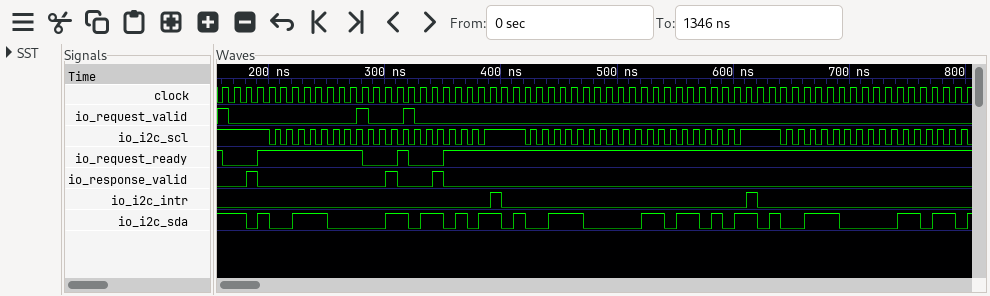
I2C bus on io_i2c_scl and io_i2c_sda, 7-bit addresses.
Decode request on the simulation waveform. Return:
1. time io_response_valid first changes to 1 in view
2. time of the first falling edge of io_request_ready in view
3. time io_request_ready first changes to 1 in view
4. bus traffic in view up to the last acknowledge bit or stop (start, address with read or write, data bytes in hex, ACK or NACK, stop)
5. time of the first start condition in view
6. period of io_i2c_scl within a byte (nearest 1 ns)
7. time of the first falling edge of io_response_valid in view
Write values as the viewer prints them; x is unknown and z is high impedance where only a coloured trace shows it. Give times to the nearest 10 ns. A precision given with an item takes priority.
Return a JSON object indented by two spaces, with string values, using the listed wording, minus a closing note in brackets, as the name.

{
  "time io_response_valid first changes to 1 in view": "180 ns",
  "time of the first falling edge of io_request_ready in view": "160 ns",
  "time io_request_ready first changes to 1 in view": "190 ns",
  "bus traffic in view up to the last acknowledge bit or stop": "start, address 1C write ACK, 6D ACK, repeated start, address 1C write ACK, 6D ACK, repeated start, address 1C write ACK",
  "time of the first start condition in view": "180 ns",
  "period of io_i2c_scl within a byte": "10 ns",
  "time of the first falling edge of io_response_valid in view": "190 ns"
}
